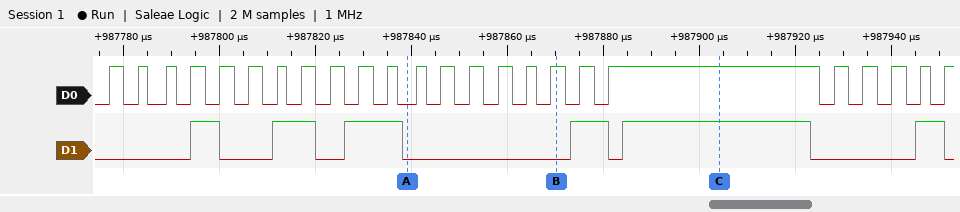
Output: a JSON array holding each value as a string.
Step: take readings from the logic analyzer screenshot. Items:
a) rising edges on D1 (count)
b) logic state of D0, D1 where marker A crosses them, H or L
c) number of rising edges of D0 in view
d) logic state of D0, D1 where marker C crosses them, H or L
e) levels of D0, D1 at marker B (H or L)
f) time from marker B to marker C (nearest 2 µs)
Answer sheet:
["6", "D0=L, D1=L", "24", "D0=H, D1=H", "D0=H, D1=L", "34 µs"]
